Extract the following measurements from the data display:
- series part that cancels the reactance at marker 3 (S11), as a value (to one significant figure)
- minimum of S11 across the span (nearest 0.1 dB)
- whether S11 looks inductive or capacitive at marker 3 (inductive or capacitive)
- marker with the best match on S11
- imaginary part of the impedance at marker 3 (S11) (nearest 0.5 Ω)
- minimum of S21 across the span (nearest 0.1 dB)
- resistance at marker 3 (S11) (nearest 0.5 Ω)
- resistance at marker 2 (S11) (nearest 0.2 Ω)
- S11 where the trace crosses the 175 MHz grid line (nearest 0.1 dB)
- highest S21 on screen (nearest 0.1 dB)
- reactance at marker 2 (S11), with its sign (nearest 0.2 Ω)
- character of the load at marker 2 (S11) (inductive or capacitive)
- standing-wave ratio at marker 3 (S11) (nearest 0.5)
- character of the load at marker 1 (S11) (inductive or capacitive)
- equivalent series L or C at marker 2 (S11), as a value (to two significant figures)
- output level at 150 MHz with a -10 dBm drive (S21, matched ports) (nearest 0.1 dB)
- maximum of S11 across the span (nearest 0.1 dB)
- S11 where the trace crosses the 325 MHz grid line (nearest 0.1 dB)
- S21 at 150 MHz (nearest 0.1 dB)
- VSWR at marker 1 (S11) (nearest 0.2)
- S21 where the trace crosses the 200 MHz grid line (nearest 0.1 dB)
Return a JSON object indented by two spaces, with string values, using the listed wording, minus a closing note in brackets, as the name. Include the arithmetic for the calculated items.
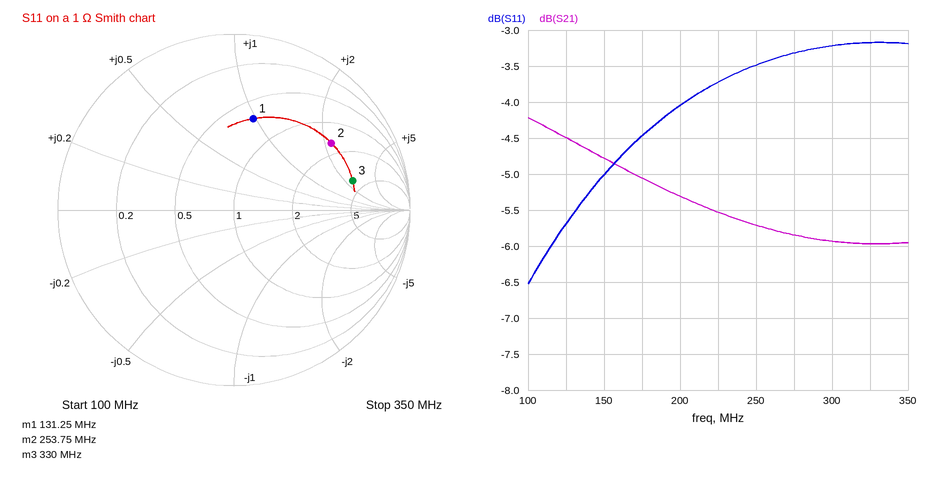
{
  "series part that cancels the reactance at marker 3 (S11), as a value": "C = 1/(2π × 330 MHz × 2.5 Ω) ≈ 193 pF, so 200 pF to one significant figure",
  "minimum of S11 across the span": "-6.5 dB",
  "whether S11 looks inductive or capacitive at marker 3": "inductive",
  "marker with the best match on S11": "marker 1",
  "imaginary part of the impedance at marker 3 (S11)": "+2.5 Ω",
  "minimum of S21 across the span": "-6.0 dB",
  "resistance at marker 3 (S11)": "4.0 Ω",
  "resistance at marker 2 (S11)": "1.6 Ω",
  "S11 where the trace crosses the 175 MHz grid line": "-4.5 dB",
  "highest S21 on screen": "-4.2 dB",
  "reactance at marker 2 (S11), with its sign": "+2.2 Ω",
  "character of the load at marker 2 (S11)": "inductive",
  "standing-wave ratio at marker 3 (S11)": "5.5",
  "character of the load at marker 1 (S11)": "inductive",
  "equivalent series L or C at marker 2 (S11), as a value": "L = 2.2 Ω/(2π × 253.75 MHz) ≈ 1.4 nH",
  "output level at 150 MHz with a -10 dBm drive (S21, matched ports)": "-10 dBm + (-4.8 dB) = -14.8 dBm",
  "maximum of S11 across the span": "-3.2 dB",
  "S11 where the trace crosses the 325 MHz grid line": "-3.2 dB",
  "S21 at 150 MHz": "-4.8 dB",
  "VSWR at marker 1 (S11)": "3.2",
  "S21 where the trace crosses the 200 MHz grid line": "-5.3 dB"
}
